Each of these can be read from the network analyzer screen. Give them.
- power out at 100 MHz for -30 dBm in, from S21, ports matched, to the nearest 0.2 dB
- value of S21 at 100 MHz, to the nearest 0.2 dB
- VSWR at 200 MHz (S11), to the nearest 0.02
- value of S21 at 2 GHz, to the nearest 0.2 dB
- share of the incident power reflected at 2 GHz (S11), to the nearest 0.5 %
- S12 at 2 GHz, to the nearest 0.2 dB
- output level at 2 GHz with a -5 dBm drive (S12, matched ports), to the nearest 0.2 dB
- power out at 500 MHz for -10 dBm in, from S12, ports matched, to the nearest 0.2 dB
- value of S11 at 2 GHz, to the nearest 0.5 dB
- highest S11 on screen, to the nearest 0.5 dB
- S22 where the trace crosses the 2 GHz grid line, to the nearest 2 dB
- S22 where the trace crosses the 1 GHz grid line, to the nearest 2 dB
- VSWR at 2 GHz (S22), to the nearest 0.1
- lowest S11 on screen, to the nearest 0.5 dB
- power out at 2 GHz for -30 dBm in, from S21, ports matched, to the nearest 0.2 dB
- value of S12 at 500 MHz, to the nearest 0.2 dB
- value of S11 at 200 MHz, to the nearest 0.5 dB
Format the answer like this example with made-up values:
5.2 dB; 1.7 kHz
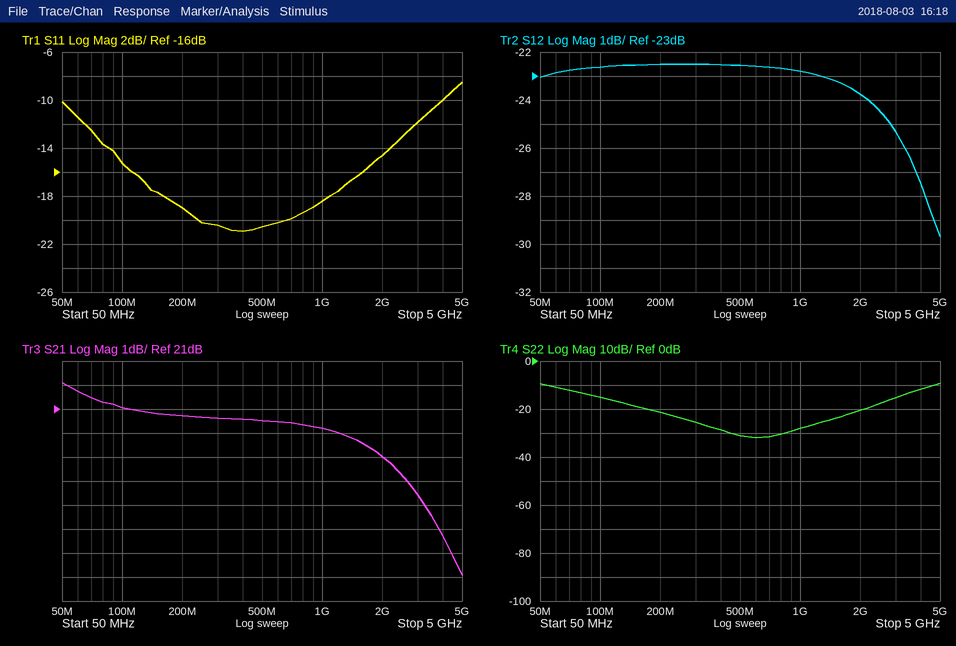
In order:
-9.0 dBm; 21.0 dB; 1.26; 19.0 dB; 3.5 %; -23.8 dB; -28.8 dBm; -32.6 dBm; -14.5 dB; -8.5 dB; -20 dB; -28 dB; 1.2; -21.0 dB; -11.0 dBm; -22.6 dB; -19.0 dB
